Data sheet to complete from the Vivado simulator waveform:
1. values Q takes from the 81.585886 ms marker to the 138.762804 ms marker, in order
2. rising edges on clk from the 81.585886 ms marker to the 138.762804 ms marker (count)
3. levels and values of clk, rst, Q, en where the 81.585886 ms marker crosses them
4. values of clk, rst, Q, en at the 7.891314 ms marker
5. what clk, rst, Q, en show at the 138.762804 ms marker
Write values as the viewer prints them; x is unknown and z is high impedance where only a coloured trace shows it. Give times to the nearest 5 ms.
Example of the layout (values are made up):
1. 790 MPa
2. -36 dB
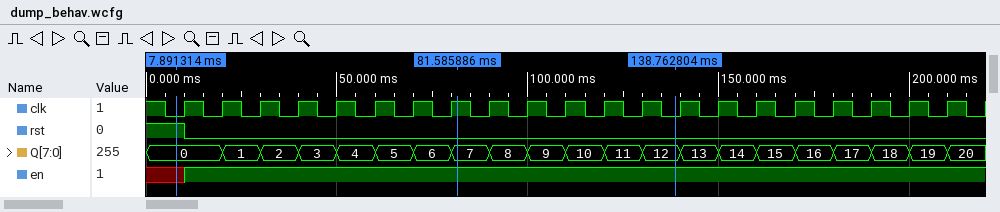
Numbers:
1. 7, 8, 9, 10, 11, 12
2. 5
3. clk=1, rst=0, Q=7, en=1
4. clk=0, rst=1, Q=0, en=x
5. clk=0, rst=0, Q=12, en=1
